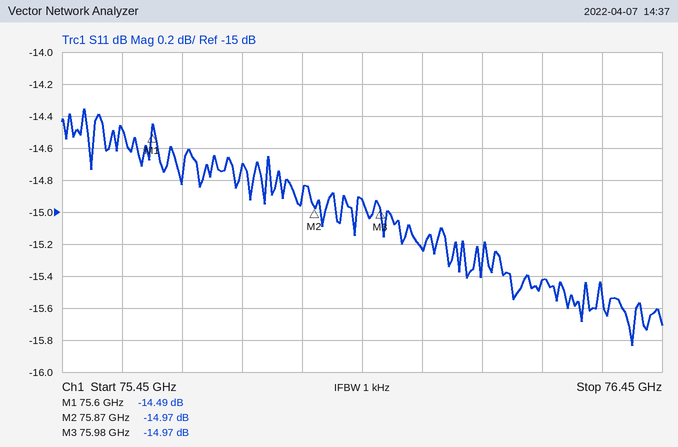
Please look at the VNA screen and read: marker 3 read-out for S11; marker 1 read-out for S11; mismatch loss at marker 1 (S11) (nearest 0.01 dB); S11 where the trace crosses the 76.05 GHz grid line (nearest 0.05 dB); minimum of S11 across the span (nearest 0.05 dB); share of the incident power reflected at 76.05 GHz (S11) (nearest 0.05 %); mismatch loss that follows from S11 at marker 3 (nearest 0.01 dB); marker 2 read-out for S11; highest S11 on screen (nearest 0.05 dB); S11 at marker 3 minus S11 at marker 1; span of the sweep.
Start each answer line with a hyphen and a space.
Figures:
- -14.97 dB
- -14.49 dB
- 0.16 dB
- -15.25 dB
- -15.85 dB
- 3.00 %
- 0.14 dB
- -14.97 dB
- -14.35 dB
- -0.48 dB
- 1 GHz
